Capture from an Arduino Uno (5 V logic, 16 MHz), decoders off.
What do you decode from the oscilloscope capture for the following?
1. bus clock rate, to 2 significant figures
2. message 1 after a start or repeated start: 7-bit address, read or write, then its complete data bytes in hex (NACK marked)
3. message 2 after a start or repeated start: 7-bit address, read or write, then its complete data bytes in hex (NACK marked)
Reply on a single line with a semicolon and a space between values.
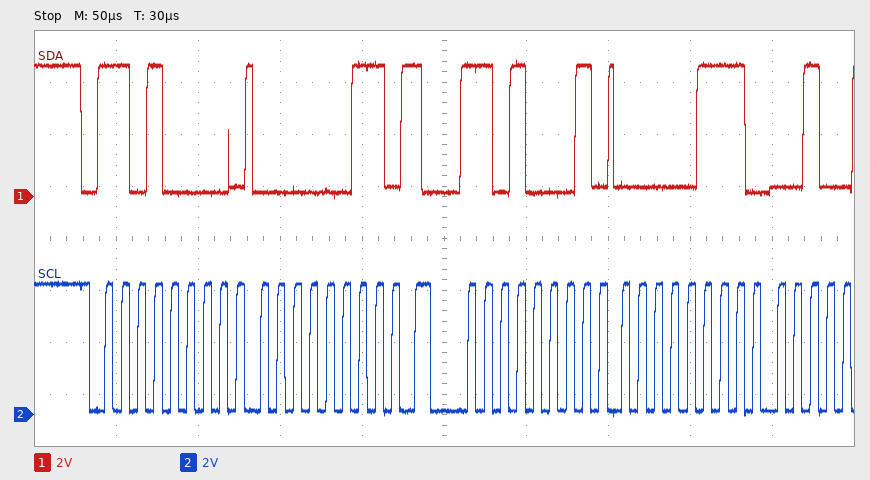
100 kHz; 0x68 write: 03; 0x68 read: 07
